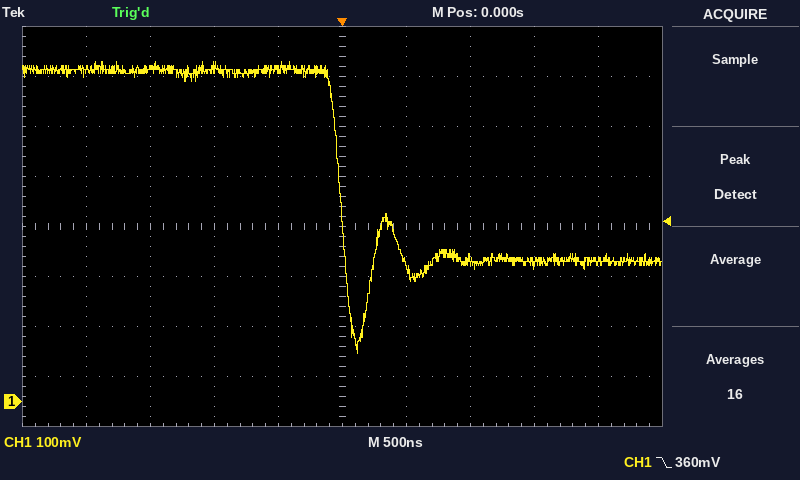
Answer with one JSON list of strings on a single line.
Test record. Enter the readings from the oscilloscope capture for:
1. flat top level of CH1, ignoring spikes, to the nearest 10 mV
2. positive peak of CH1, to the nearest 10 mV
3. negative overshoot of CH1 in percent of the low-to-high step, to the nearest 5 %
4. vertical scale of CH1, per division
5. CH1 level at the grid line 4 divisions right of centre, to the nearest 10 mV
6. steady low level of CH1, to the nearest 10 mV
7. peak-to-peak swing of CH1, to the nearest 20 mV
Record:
["660 mV", "680 mV", "50 %", "100 mV", "280 mV", "280 mV", "580 mV"]
